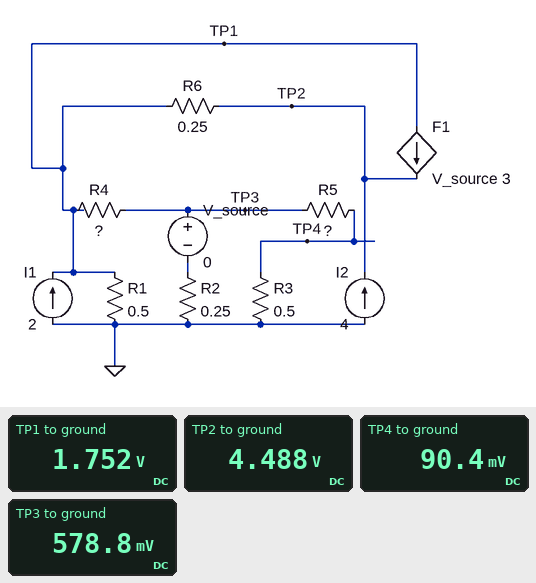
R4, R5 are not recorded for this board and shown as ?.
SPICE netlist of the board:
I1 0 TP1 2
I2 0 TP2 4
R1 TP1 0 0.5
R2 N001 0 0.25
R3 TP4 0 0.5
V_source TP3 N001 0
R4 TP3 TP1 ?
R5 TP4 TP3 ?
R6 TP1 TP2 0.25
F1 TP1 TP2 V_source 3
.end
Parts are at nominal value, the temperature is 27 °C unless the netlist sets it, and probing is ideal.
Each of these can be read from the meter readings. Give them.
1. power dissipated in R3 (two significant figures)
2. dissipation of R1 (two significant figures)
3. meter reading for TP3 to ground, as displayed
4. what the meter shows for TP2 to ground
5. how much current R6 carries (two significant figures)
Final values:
16 mW
6.1 W
578.8 mV
4.488 V
11 A
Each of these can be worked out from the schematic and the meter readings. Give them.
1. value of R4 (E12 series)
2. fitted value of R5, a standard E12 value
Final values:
0.47 Ω
2.7 Ω
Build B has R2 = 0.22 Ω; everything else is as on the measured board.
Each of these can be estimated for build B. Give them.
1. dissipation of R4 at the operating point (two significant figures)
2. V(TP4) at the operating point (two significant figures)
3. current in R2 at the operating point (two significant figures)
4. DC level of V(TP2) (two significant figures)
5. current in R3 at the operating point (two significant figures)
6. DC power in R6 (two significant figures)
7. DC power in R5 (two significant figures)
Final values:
3.1 W
82 mV
2.4 A
4.5 V
160 mA
31 W
73 mW
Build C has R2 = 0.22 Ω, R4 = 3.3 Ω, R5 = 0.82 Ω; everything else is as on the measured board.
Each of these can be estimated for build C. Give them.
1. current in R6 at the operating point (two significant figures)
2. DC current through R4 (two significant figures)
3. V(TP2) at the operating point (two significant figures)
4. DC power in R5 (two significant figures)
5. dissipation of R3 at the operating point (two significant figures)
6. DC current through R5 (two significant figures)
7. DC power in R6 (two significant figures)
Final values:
5.9 A
750 mA
4.1 V
9.5 mW
5.8 mW
110 mA
8.8 W
